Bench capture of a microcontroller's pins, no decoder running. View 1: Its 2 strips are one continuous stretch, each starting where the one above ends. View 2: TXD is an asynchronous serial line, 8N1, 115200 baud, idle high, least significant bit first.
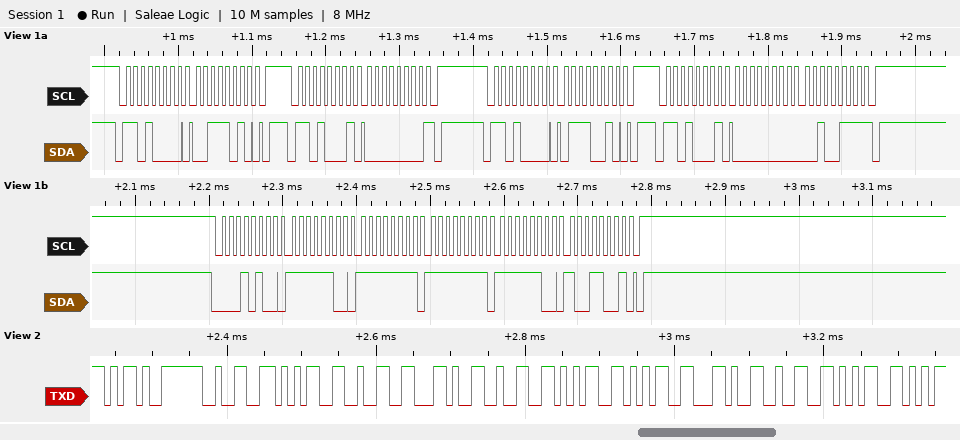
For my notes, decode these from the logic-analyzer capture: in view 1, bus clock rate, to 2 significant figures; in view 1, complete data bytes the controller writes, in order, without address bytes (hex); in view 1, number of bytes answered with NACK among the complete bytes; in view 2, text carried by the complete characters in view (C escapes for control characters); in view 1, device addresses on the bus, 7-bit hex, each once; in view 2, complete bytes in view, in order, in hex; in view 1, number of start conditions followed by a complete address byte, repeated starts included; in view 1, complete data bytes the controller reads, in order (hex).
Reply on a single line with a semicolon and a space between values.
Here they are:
100 kHz; 3A 72 FC FF FF FC 99; 2; "-252,255,25"; 0x68 0x0A; 2D 32 35 32 2C 32 35 35 2C 32 35; 5; 00 00 27
